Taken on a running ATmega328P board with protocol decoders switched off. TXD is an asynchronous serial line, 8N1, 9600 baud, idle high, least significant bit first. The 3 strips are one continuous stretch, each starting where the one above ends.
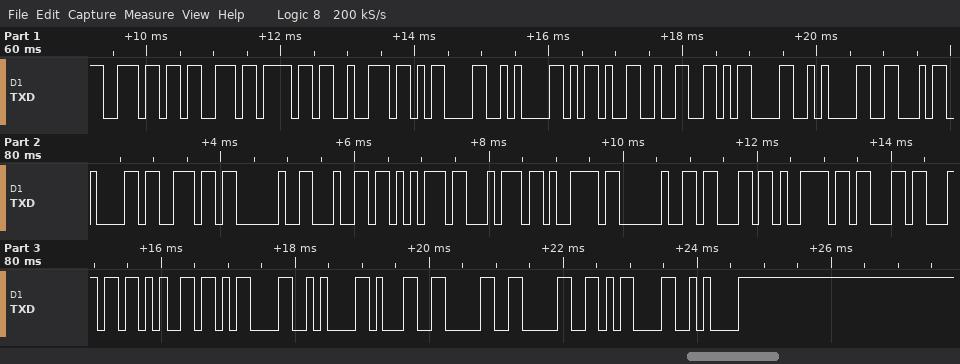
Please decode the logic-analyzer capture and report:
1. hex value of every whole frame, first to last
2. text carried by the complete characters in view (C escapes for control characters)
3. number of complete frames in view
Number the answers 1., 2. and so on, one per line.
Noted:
1. 6E 73 6F 72 0D 0A 2D 32 0D 0A 46 61 6E 20 64 75 74 79 20 63 79 63 6C 65 0D 0A 31 30 30 0D 0A
2. "nsor\r\n-2\r\nFan duty cycle\r\n100\r\n"
3. 31
